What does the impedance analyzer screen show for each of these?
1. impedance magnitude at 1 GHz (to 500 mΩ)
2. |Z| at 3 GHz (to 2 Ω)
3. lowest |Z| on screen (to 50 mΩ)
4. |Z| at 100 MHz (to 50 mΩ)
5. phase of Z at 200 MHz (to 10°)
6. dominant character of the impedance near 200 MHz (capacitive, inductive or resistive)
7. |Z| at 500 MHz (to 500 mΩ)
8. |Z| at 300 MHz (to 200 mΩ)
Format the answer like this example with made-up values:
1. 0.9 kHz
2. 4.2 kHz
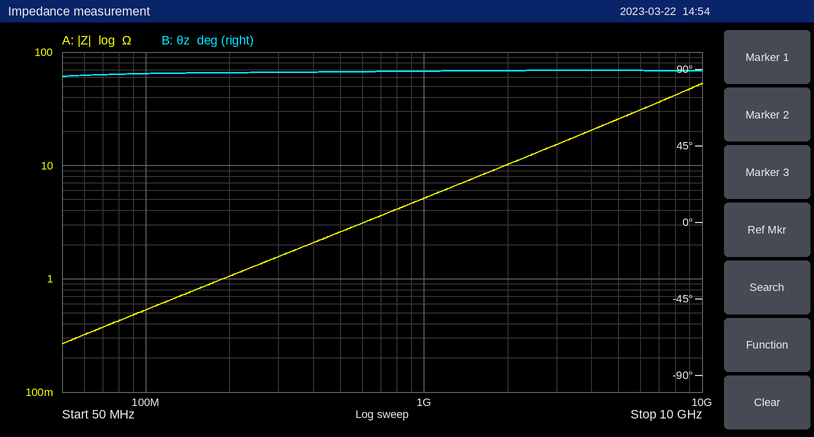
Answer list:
1. 5.0 Ω
2. 16 Ω
3. 250 mΩ
4. 550 mΩ
5. 90°
6. inductive
7. 2.5 Ω
8. 1.6 Ω
